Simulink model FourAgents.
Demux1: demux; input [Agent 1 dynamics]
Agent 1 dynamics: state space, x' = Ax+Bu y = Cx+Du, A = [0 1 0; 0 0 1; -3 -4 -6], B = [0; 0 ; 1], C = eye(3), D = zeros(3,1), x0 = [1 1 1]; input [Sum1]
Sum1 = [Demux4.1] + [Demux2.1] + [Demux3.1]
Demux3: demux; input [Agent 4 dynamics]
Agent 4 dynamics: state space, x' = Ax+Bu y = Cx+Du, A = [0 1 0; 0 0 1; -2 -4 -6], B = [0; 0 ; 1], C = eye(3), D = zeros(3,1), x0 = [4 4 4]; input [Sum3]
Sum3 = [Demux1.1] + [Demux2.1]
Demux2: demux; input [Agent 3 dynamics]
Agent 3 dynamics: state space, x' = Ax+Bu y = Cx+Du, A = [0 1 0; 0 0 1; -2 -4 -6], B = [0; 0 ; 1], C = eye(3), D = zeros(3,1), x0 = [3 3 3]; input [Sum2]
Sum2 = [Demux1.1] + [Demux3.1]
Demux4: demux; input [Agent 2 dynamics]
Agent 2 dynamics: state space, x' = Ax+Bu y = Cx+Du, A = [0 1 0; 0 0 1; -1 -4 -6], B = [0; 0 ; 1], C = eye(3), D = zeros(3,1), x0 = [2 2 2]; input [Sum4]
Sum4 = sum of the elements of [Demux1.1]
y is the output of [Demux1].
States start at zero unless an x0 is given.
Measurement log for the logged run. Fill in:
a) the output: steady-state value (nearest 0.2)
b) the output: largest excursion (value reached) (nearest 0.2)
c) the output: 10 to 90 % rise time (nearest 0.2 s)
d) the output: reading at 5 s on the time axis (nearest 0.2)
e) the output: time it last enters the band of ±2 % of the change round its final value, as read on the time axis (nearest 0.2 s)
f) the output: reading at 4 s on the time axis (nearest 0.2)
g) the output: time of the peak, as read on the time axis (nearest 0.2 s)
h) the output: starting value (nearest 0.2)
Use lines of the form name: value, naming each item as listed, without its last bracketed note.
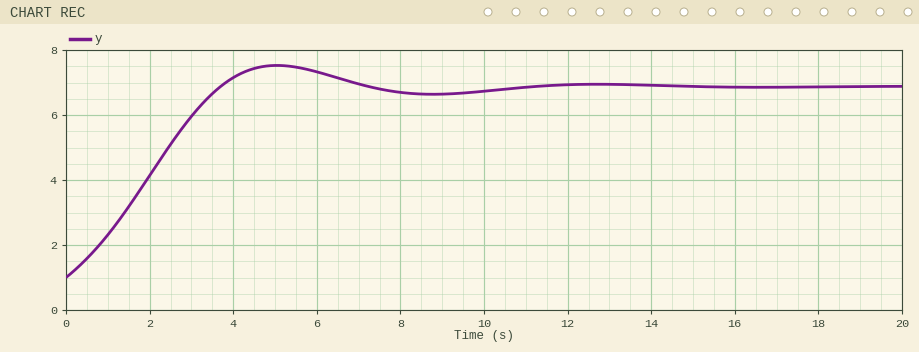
the output: steady-state value: 6.8
the output: largest excursion (value reached): 7.6
the output: 10 to 90 % rise time: 2.8 s
the output: reading at 5 s on the time axis: 7.6
the output: time it last enters the band of ±2 % of the change round its final value, as read on the time axis: 10.2 s
the output: reading at 4 s on the time axis: 7.2
the output: time of the peak, as read on the time axis: 5.0 s
the output: starting value: 1.0
